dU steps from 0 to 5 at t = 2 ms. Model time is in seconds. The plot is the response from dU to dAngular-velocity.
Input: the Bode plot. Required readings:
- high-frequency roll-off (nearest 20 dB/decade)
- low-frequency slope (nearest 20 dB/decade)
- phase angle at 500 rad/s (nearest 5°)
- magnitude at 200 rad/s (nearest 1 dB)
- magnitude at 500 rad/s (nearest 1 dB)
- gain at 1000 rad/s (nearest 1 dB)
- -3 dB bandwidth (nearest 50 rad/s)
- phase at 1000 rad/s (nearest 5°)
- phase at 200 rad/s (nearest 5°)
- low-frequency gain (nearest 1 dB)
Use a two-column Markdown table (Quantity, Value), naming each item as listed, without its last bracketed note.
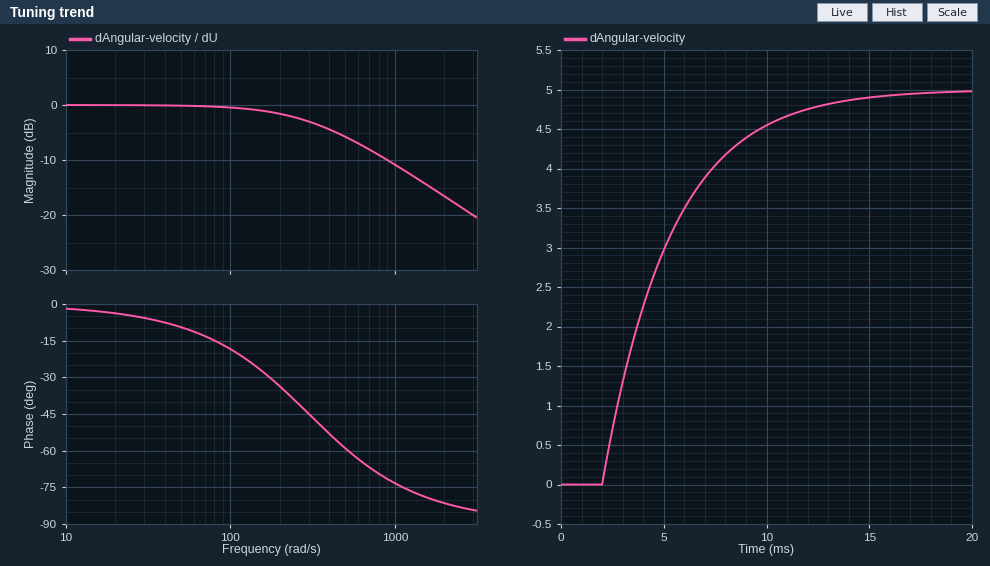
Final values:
| Quantity | Value |
|---|---|
| high-frequency roll-off | -20 dB/decade |
| low-frequency slope | 0 dB/decade |
| phase angle at 500 rad/s | -60° |
| magnitude at 200 rad/s | -2 dB |
| magnitude at 500 rad/s | -6 dB |
| gain at 1000 rad/s | -11 dB |
| -3 dB bandwidth | 300 rad/s |
| phase at 1000 rad/s | -75° |
| phase at 200 rad/s | -35° |
| low-frequency gain | 0 dB |
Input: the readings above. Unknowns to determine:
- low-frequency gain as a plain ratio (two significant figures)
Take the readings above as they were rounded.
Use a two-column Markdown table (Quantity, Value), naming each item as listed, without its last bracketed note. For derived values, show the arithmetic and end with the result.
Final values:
| Quantity | Value |
|---|---|
| low-frequency gain as a plain ratio | 10^(0 / 20) = 1.0 |
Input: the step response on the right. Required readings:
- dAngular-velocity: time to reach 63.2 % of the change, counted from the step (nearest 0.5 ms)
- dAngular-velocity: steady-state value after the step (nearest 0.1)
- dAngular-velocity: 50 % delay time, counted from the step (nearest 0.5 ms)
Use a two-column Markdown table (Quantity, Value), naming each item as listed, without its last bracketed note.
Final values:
| Quantity | Value |
|---|---|
| dAngular-velocity: time to reach 63.2 % of the change, counted from the step | 3.5 ms |
| dAngular-velocity: steady-state value after the step | 5.0 |
| dAngular-velocity: 50 % delay time, counted from the step | 2.5 ms |
